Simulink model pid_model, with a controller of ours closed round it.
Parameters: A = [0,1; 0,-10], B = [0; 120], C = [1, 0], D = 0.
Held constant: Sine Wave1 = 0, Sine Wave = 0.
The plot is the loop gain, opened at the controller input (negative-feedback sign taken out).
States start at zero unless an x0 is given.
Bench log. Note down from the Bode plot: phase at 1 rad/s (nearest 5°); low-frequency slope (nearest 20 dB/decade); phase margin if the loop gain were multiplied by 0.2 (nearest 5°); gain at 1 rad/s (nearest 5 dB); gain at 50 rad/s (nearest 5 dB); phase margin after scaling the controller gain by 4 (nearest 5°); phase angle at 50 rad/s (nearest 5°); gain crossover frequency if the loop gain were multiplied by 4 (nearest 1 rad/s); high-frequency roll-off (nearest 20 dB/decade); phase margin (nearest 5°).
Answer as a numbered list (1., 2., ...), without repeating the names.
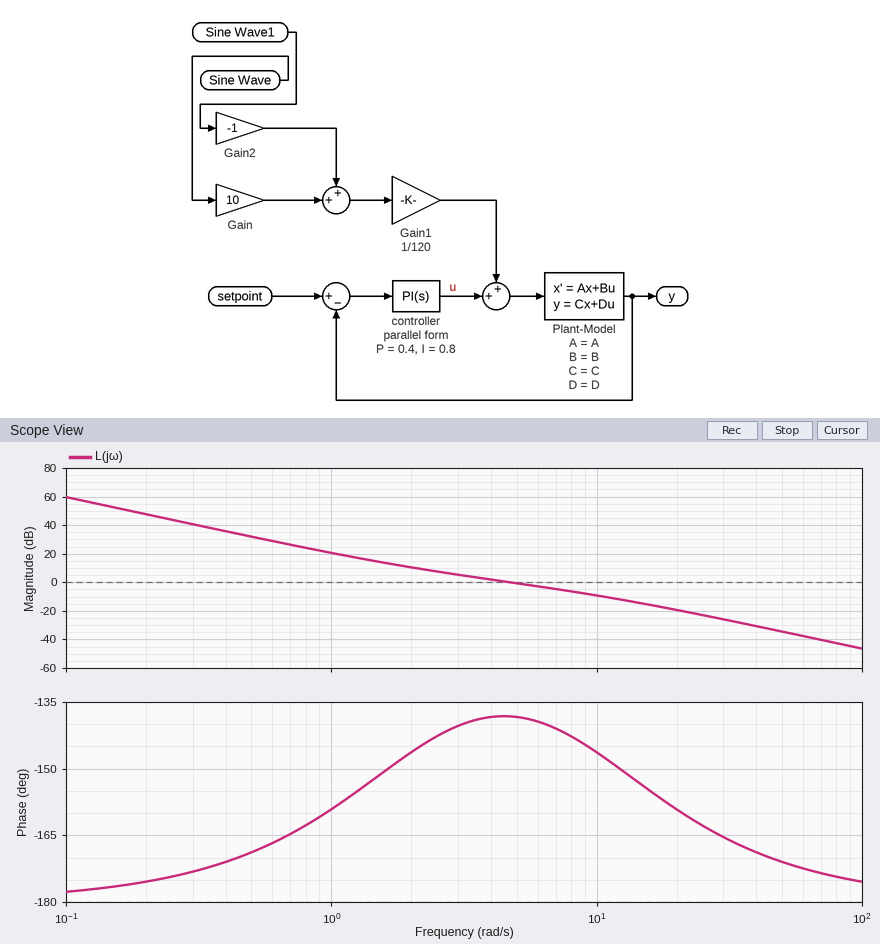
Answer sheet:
1. -160°
2. -40 dB/decade
3. 30°
4. 20 dB
5. -35 dB
6. 30°
7. -170°
8. 12 rad/s
9. -40 dB/decade
10. 40°
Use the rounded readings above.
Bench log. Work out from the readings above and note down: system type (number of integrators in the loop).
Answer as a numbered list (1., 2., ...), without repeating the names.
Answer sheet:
1. 2
